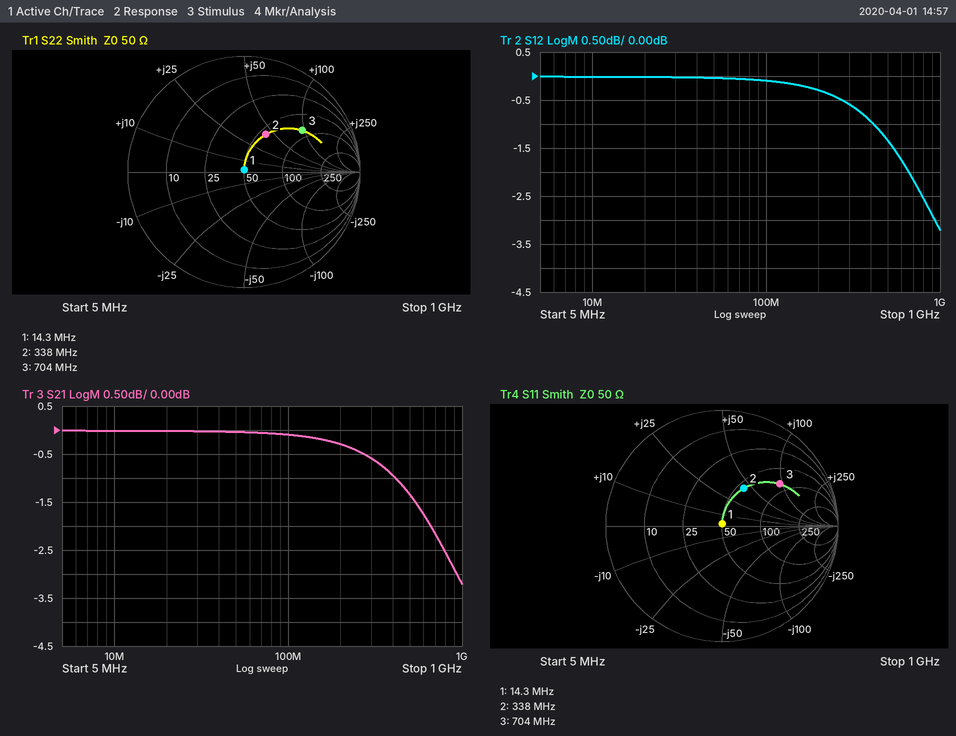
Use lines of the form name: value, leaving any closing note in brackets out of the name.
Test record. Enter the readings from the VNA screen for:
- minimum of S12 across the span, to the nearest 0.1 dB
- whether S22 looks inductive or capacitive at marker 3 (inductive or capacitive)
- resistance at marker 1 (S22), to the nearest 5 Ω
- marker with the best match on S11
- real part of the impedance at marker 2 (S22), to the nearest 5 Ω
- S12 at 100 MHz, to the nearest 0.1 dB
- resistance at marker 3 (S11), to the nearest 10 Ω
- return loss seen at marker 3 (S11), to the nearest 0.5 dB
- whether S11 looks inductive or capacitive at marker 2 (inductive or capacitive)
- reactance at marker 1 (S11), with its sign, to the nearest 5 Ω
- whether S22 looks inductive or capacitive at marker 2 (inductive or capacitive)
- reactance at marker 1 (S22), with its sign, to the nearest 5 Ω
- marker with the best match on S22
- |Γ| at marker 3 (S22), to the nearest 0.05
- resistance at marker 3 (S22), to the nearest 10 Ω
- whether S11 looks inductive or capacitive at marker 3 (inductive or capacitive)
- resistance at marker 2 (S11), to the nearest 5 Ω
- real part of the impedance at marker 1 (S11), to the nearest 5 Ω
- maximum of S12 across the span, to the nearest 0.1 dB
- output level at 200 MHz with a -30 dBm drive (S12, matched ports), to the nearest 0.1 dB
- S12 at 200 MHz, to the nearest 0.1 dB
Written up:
minimum of S12 across the span, to the nearest 0.1 dB: -3.2 dB
whether S22 looks inductive or capacitive at marker 3: inductive
resistance at marker 1 (S22), to the nearest 5 Ω: 50 Ω
marker with the best match on S11: marker 1
real part of the impedance at marker 2 (S22), to the nearest 5 Ω: 55 Ω
S12 at 100 MHz, to the nearest 0.1 dB: -0.1 dB
resistance at marker 3 (S11), to the nearest 10 Ω: 80 Ω
return loss seen at marker 3 (S11), to the nearest 0.5 dB: 4.0 dB
whether S11 looks inductive or capacitive at marker 2: inductive
reactance at marker 1 (S11), with its sign, to the nearest 5 Ω: 0 Ω
whether S22 looks inductive or capacitive at marker 2: inductive
reactance at marker 1 (S22), with its sign, to the nearest 5 Ω: 0 Ω
marker with the best match on S22: marker 1
|Γ| at marker 3 (S22), to the nearest 0.05: 0.60
resistance at marker 3 (S22), to the nearest 10 Ω: 80 Ω
whether S11 looks inductive or capacitive at marker 3: inductive
resistance at marker 2 (S11), to the nearest 5 Ω: 55 Ω
real part of the impedance at marker 1 (S11), to the nearest 5 Ω: 50 Ω
maximum of S12 across the span, to the nearest 0.1 dB: 0.0 dB
output level at 200 MHz with a -30 dBm drive (S12, matched ports), to the nearest 0.1 dB: -30.3 dBm
S12 at 200 MHz, to the nearest 0.1 dB: -0.3 dB
